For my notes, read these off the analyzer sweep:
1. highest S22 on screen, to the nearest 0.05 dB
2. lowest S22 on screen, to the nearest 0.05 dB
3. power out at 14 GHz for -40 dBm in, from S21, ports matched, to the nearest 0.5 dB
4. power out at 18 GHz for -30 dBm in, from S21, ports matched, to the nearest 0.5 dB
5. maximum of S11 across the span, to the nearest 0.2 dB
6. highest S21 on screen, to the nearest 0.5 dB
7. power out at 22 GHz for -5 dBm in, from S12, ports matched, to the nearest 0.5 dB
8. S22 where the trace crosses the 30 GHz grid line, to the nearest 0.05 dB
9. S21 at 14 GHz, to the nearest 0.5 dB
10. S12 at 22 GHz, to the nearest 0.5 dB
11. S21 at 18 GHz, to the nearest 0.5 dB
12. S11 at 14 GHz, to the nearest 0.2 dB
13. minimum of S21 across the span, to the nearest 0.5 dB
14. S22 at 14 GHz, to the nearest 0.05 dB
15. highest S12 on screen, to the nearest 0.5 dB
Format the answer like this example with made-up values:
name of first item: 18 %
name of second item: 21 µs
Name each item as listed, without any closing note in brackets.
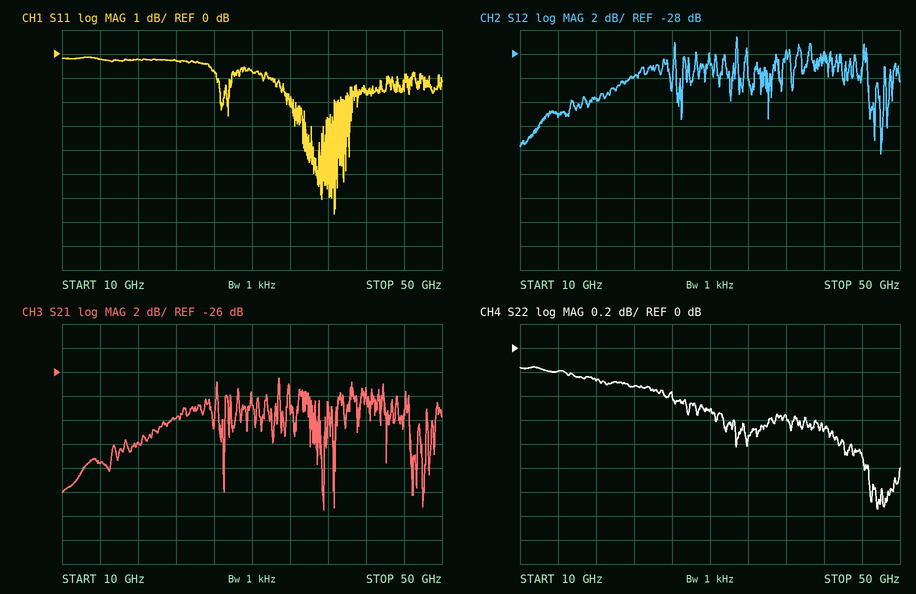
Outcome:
highest S22 on screen, to the nearest 0.05 dB: -0.15 dB
lowest S22 on screen, to the nearest 0.05 dB: -1.35 dB
power out at 14 GHz for -40 dBm in, from S21, ports matched, to the nearest 0.5 dB: -73.5 dBm
power out at 18 GHz for -30 dBm in, from S21, ports matched, to the nearest 0.5 dB: -62.0 dBm
maximum of S11 across the span, to the nearest 0.2 dB: -0.2 dB
highest S21 on screen, to the nearest 0.5 dB: -26.5 dB
power out at 22 GHz for -5 dBm in, from S12, ports matched, to the nearest 0.5 dB: -35.0 dBm
S22 where the trace crosses the 30 GHz grid line, to the nearest 0.05 dB: -0.50 dB
S21 at 14 GHz, to the nearest 0.5 dB: -33.5 dB
S12 at 22 GHz, to the nearest 0.5 dB: -30.0 dB
S21 at 18 GHz, to the nearest 0.5 dB: -32.0 dB
S11 at 14 GHz, to the nearest 0.2 dB: -0.2 dB
minimum of S21 across the span, to the nearest 0.5 dB: -37.5 dB
S22 at 14 GHz, to the nearest 0.05 dB: -0.20 dB
highest S12 on screen, to the nearest 0.5 dB: -26.5 dB
